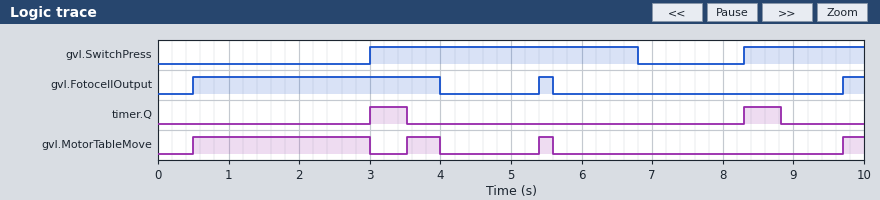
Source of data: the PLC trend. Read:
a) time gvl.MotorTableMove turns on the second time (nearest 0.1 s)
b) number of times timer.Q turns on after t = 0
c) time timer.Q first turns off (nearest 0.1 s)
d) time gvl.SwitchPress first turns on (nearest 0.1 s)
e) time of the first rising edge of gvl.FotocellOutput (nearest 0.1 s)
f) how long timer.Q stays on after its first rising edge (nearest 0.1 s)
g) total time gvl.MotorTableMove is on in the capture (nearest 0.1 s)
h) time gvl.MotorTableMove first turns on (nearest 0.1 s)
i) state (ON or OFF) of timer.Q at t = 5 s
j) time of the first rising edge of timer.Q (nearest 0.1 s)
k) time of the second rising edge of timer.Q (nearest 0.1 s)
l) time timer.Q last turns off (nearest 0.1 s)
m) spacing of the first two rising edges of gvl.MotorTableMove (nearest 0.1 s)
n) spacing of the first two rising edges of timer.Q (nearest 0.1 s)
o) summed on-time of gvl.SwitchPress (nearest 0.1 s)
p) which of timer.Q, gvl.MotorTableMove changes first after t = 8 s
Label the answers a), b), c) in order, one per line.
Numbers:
a) 3.5 s
b) 2
c) 3.5 s
d) 3.0 s
e) 0.5 s
f) 0.5 s
g) 3.5 s
h) 0.5 s
i) OFF
j) 3.0 s
k) 8.3 s
l) 8.8 s
m) 3.0 s
n) 5.3 s
o) 5.5 s
p) timer.Q
